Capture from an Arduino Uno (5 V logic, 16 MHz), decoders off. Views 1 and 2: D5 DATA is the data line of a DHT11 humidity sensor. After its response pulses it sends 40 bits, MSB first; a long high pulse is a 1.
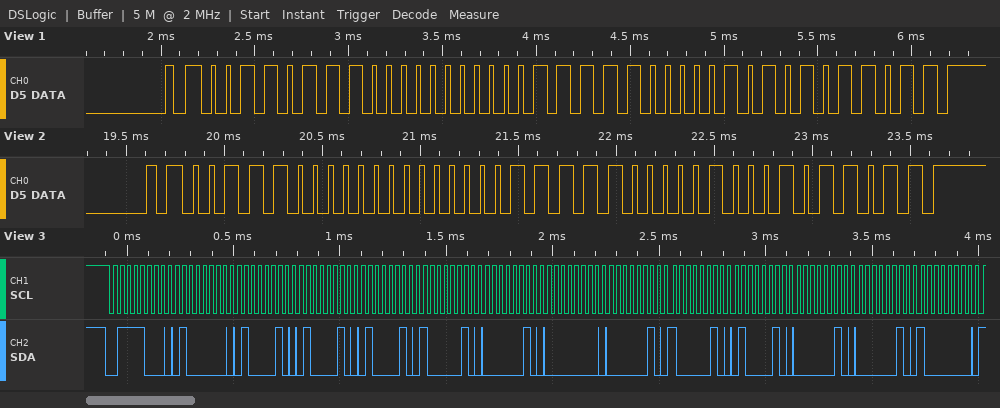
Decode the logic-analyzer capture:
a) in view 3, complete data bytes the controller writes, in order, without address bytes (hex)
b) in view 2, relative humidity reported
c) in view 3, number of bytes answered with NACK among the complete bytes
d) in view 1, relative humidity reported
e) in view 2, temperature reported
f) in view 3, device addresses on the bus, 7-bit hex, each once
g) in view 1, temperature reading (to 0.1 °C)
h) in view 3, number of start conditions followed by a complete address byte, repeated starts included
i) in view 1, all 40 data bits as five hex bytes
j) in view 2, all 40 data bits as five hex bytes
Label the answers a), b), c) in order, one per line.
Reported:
a) 40 42 42 42 82 02 00 02 82 42 02 02 80
b) 56 %
c) 0
d) 55 %
e) 31.4 °C
f) 0x3C
g) 31.5 °C
h) 1
i) 37 00 1F 05 5B
j) 38 00 1F 04 5B
